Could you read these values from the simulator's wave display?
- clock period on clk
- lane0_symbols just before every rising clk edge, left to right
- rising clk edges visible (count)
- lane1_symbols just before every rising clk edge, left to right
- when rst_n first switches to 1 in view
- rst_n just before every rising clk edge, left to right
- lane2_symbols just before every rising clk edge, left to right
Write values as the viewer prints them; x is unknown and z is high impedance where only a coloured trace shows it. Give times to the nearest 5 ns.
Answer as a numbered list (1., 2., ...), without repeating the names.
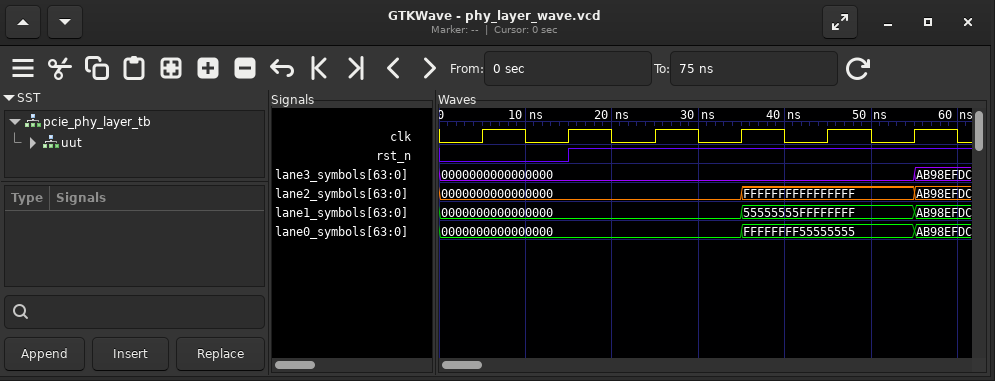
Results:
1. 10 ns
2. 0000000000000000, 0000000000000000, 0000000000000000, 0000000000000000, FFFFFFFF55555555, FFFFFFFF55555555
3. 6
4. 0000000000000000, 0000000000000000, 0000000000000000, 0000000000000000, 55555555FFFFFFFF, 55555555FFFFFFFF
5. 15 ns
6. 0 0 1 1 1 1
7. 0000000000000000, 0000000000000000, 0000000000000000, 0000000000000000, FFFFFFFFFFFFFFFF, FFFFFFFFFFFFFFFF
